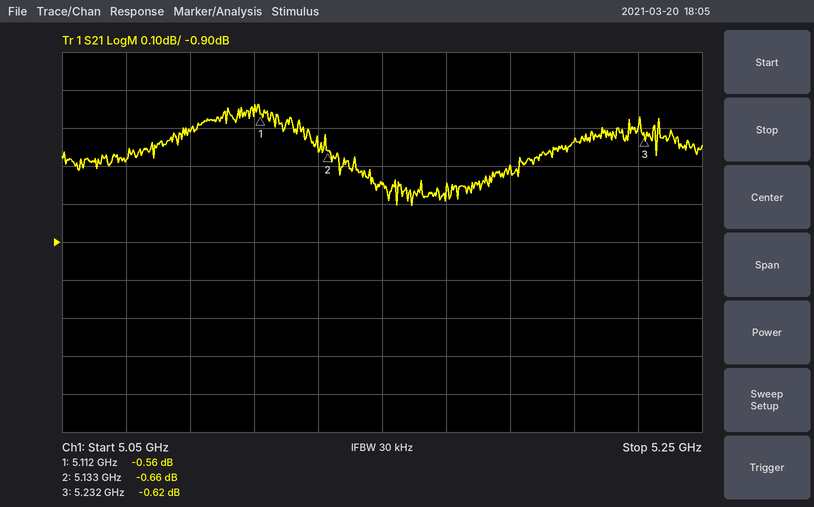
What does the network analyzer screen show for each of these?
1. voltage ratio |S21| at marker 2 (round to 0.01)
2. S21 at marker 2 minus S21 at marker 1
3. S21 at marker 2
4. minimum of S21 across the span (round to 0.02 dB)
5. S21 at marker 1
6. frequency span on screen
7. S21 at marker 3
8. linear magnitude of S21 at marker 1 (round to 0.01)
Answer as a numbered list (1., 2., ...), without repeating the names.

1. 0.93
2. -0.10 dB
3. -0.66 dB
4. -0.80 dB
5. -0.56 dB
6. 200 MHz
7. -0.62 dB
8. 0.94
